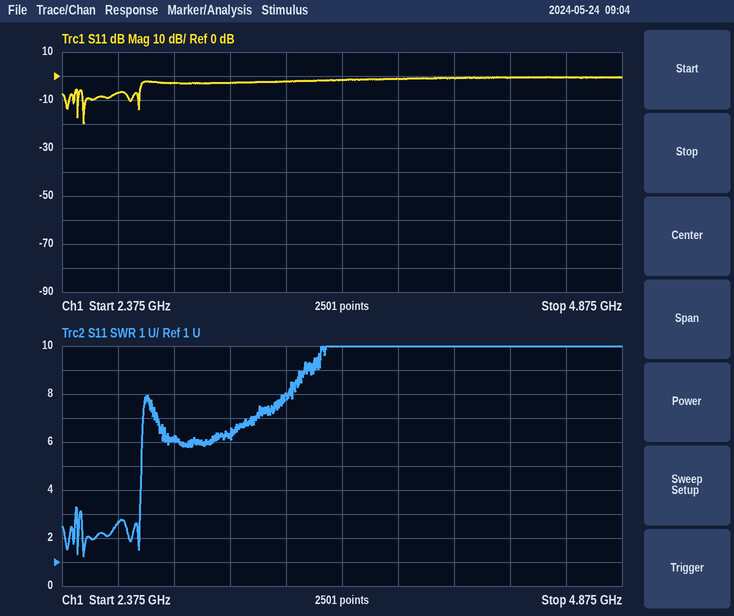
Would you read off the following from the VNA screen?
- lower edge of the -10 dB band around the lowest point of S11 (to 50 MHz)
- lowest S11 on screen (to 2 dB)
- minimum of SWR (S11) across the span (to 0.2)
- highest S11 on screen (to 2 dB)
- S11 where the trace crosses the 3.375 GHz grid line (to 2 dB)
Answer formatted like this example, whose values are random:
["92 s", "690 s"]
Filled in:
["2.45 GHz", "-20 dB", "1.2", "0 dB", "-2 dB"]
